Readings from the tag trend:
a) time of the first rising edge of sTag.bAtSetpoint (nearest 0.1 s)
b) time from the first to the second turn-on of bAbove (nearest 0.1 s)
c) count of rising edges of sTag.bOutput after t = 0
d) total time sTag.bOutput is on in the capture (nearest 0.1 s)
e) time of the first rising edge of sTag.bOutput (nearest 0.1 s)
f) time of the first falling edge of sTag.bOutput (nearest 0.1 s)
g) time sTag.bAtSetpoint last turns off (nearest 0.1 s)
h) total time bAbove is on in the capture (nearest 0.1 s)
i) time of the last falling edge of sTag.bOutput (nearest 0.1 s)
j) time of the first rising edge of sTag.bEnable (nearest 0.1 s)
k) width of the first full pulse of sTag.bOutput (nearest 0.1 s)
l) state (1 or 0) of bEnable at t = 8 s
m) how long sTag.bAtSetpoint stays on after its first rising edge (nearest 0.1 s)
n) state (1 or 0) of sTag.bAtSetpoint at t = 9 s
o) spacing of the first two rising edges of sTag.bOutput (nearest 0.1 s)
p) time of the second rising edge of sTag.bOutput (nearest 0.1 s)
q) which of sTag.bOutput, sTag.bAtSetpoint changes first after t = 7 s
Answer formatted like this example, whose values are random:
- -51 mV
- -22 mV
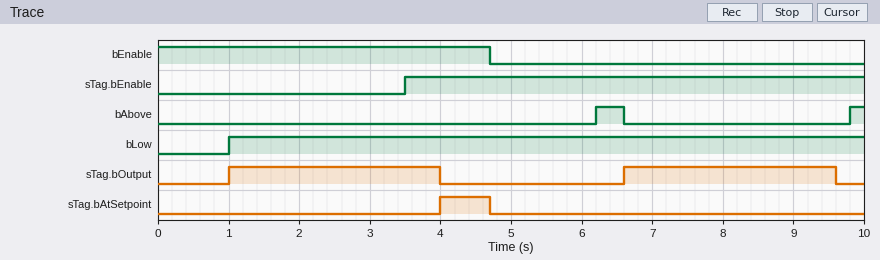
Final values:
- 4.0 s
- 3.6 s
- 2
- 6.0 s
- 1.0 s
- 4.0 s
- 4.7 s
- 0.6 s
- 9.6 s
- 3.5 s
- 3.0 s
- 0
- 0.7 s
- 0
- 5.6 s
- 6.6 s
- sTag.bOutput
